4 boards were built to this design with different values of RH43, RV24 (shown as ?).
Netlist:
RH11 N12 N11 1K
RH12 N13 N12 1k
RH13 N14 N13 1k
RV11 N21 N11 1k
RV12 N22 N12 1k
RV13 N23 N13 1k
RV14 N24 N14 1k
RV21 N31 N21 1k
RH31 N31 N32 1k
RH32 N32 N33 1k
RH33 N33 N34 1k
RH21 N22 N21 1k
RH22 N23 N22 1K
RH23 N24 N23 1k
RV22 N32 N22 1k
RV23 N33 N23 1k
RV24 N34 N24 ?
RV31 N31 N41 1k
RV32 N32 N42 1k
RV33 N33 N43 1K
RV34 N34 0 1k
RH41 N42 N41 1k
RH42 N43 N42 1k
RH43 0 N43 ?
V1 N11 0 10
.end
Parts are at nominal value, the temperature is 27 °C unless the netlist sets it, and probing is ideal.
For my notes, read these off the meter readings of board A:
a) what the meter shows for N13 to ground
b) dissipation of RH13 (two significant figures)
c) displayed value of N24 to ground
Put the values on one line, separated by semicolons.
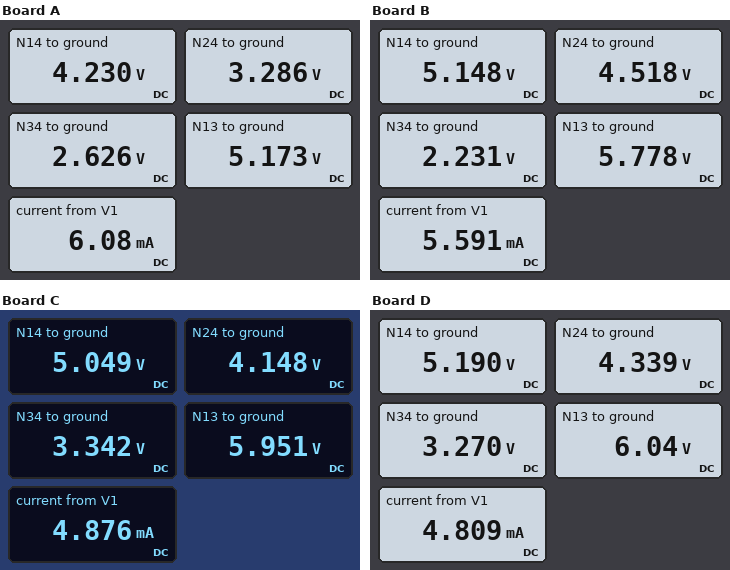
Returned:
5.173 V; 890 µW; 3.286 V
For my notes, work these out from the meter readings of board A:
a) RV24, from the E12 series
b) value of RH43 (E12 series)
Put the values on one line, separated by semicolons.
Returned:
330 Ω; 470 Ω
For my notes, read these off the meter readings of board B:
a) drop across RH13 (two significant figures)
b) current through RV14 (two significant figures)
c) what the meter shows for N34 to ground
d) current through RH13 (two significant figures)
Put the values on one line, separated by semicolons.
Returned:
630 mV; 630 µA; 2.231 V; 630 µA
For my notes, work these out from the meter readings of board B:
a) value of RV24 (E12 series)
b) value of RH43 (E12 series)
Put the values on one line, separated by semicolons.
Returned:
2.2 kΩ; 560 Ω
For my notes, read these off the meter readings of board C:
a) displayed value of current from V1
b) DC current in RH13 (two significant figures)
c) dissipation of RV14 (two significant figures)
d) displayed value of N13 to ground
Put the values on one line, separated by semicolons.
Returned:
4.876 mA; 900 µA; 810 µW; 5.951 V
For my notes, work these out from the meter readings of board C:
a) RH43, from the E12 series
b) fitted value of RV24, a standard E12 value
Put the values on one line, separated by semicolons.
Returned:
2.7 kΩ; 390 Ω
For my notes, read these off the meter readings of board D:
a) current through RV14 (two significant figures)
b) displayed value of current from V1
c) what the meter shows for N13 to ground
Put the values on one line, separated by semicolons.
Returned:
850 µA; 4.809 mA; 6.04 V
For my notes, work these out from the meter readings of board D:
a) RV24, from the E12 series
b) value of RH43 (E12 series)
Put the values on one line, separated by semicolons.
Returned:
560 Ω; 2.7 kΩ
